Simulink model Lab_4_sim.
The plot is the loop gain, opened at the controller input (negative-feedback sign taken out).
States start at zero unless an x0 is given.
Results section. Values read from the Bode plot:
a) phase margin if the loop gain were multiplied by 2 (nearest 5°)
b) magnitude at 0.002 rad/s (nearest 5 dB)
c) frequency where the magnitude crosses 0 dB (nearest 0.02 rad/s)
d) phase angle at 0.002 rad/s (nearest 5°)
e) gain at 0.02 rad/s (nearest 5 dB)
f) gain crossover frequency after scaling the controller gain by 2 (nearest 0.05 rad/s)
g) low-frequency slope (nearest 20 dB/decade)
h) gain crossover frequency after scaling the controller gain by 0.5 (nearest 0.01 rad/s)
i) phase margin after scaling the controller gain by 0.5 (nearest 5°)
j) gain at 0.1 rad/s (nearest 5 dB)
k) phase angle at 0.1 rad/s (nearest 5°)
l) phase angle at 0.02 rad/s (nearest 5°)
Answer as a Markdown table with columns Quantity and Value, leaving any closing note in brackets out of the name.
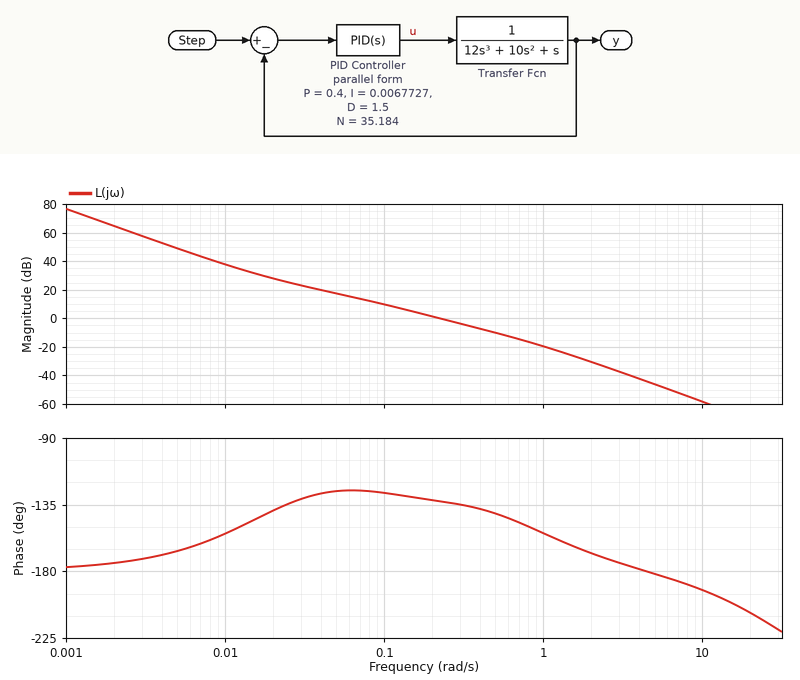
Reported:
| Quantity | Value |
|---|---|
| phase margin if the loop gain were multiplied by 2 | 45° |
| magnitude at 0.002 rad/s | 65 dB |
| frequency where the magnitude crosses 0 dB | 0.22 rad/s |
| phase angle at 0.002 rad/s | -175° |
| gain at 0.02 rad/s | 30 dB |
| gain crossover frequency after scaling the controller gain by 2 | 0.35 rad/s |
| low-frequency slope | -40 dB/decade |
| gain crossover frequency after scaling the controller gain by 0.5 | 0.14 rad/s |
| phase margin after scaling the controller gain by 0.5 | 50° |
| gain at 0.1 rad/s | 10 dB |
| phase angle at 0.1 rad/s | -125° |
| phase angle at 0.02 rad/s | -140° |
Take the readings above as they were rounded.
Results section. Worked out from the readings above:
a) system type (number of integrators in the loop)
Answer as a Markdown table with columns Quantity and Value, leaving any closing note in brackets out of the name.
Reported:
| Quantity | Value |
|---|---|
| system type | 2 |
